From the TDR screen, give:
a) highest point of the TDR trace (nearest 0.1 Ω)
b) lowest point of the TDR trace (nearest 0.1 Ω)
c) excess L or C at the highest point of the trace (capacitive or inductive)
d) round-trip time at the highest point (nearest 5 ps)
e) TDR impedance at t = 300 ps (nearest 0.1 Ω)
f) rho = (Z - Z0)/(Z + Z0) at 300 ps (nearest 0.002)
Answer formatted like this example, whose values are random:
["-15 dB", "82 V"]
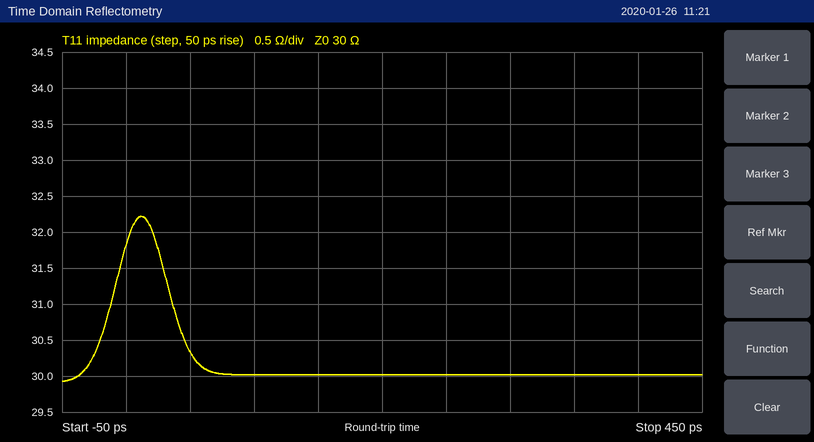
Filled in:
["32.2 Ω", "29.9 Ω", "inductive", "10 ps", "30.0 Ω", "0.000"]
